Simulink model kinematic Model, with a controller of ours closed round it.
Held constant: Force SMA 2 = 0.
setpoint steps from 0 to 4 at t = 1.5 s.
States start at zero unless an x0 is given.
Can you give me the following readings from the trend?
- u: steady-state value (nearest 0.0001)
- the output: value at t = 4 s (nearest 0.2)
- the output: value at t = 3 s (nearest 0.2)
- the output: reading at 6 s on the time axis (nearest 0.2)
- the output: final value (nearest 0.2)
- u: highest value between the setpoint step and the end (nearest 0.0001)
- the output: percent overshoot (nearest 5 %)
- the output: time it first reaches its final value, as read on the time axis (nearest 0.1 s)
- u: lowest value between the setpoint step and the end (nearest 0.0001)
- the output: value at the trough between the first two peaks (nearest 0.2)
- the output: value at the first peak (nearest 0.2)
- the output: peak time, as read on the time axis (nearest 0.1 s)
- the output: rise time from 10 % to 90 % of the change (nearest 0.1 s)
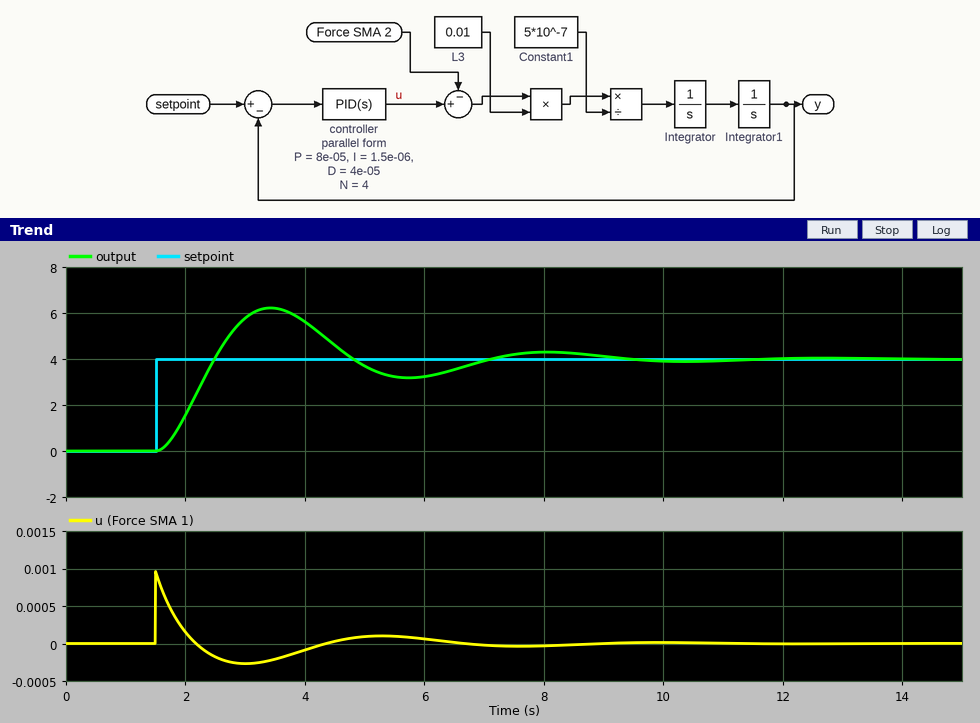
0.0000
5.6
5.8
3.2
4.0
0.0010
55 %
2.5 s
-0.0003
3.2
6.2
3.4 s
0.7 s
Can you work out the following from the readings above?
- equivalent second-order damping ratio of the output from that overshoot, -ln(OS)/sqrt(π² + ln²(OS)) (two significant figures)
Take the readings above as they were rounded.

0.19
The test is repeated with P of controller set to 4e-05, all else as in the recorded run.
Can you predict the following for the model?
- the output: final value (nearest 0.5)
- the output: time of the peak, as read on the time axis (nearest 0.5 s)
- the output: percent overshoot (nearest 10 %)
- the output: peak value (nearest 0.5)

4.0
4.0 s
40 %
5.5
